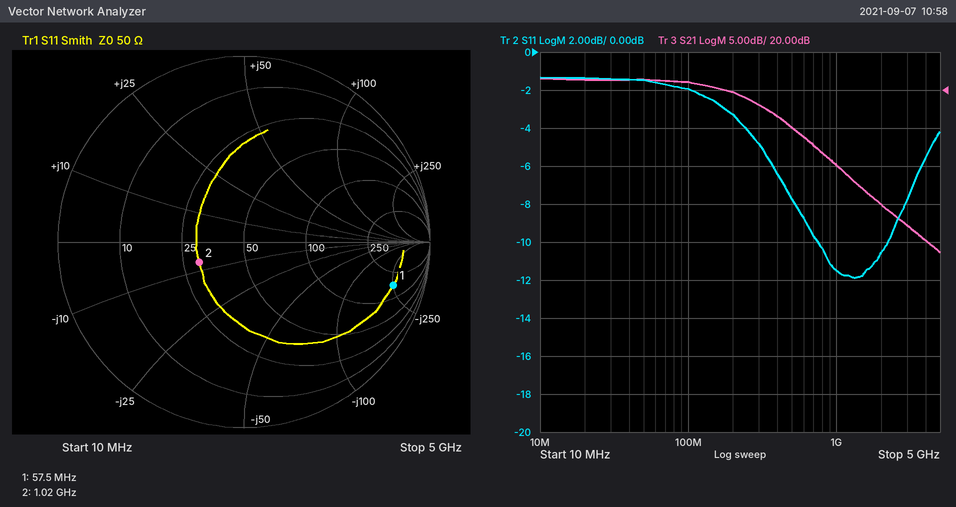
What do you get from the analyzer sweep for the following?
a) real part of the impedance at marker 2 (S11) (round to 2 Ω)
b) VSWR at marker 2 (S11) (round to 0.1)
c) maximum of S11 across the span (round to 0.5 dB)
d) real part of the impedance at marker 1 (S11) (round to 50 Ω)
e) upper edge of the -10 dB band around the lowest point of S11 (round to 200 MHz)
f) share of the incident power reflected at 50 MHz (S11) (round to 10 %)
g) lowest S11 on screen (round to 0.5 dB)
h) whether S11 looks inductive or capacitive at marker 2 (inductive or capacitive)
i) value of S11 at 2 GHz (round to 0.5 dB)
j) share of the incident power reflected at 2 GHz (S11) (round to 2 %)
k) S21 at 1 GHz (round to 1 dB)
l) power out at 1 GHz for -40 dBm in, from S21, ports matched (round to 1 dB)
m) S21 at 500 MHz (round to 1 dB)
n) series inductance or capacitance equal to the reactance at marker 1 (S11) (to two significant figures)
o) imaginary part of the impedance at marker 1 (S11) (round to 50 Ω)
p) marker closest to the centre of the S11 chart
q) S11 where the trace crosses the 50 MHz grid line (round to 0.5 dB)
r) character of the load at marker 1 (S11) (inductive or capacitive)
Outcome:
30 Ω
1.7
-1.5 dB
150 Ω
2.2 GHz
70 %
-12.0 dB
capacitive
-10.5 dB
8 %
10 dB
-30 dBm
15 dB
11 pF
-250 Ω
marker 2
-1.5 dB
capacitive
